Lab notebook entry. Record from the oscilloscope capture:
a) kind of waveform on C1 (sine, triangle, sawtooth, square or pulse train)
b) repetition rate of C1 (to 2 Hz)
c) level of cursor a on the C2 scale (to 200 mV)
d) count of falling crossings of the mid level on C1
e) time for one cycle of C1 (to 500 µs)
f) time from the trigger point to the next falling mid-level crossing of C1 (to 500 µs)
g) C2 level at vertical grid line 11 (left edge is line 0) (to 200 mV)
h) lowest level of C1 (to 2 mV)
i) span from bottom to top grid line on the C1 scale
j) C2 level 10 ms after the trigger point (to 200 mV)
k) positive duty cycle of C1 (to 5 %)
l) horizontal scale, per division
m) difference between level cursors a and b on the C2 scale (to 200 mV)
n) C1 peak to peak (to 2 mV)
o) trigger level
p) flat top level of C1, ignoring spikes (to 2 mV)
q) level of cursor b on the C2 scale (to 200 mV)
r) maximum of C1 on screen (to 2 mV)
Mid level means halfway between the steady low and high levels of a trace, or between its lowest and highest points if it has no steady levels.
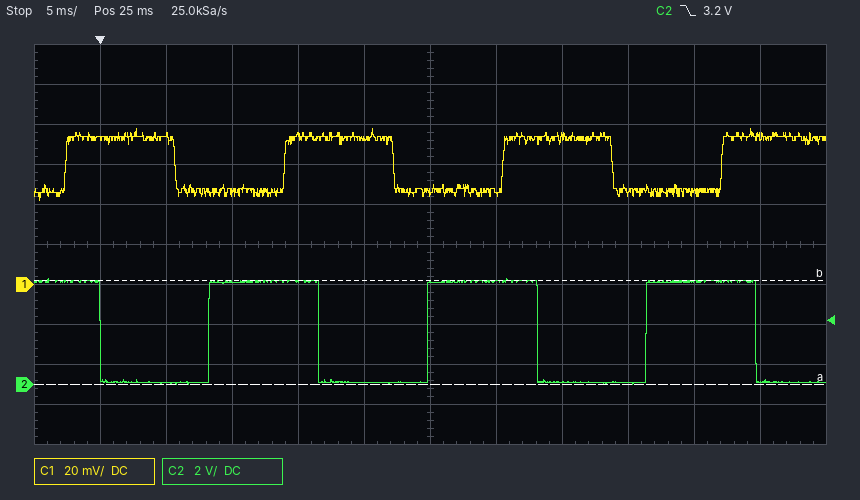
square
60 Hz
0.0 V
3
16.5 ms
5.5 ms
200 mV
42 mV
200 mV
5.2 V
50 %
5 ms
5.2 V
36 mV
3.2 V
74 mV
5.2 V
78 mV
